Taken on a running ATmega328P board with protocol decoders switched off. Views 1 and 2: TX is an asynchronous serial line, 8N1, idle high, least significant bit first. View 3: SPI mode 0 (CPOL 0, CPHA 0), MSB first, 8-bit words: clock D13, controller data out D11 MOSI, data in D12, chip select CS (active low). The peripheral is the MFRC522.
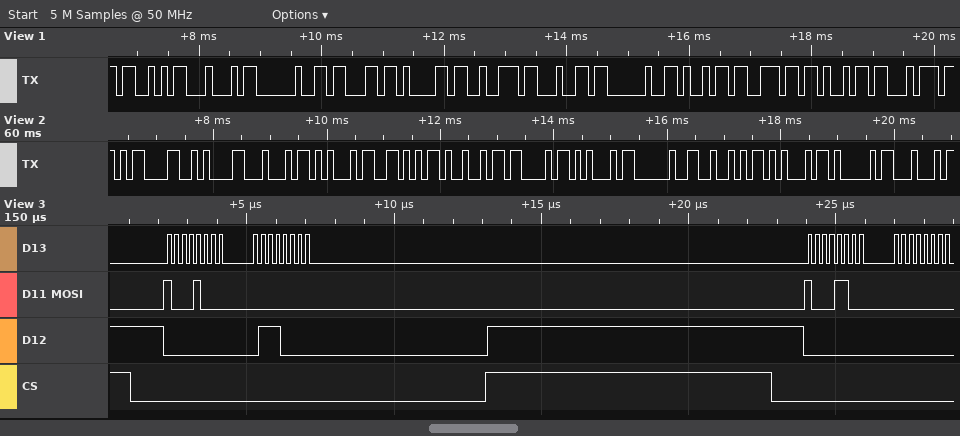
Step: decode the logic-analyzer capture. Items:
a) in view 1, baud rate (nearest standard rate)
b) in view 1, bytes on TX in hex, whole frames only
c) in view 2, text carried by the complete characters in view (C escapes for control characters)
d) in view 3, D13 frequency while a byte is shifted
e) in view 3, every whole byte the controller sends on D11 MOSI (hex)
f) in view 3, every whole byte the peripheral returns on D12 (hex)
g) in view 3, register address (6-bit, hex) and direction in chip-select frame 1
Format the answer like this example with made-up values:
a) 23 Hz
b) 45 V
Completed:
a) 9600 baud
b) 0x53 0x44 0x20 0x63 0x61 0x72 0x64 0x20 0x69 0x6E 0x69 0x74
c) "\r\nDEVICE READ"
d) 4 MHz
e) 0x88 0x00 0x8C 0x00
f) 0x00 0x70 0x00 0x00
g) 0x04 read
